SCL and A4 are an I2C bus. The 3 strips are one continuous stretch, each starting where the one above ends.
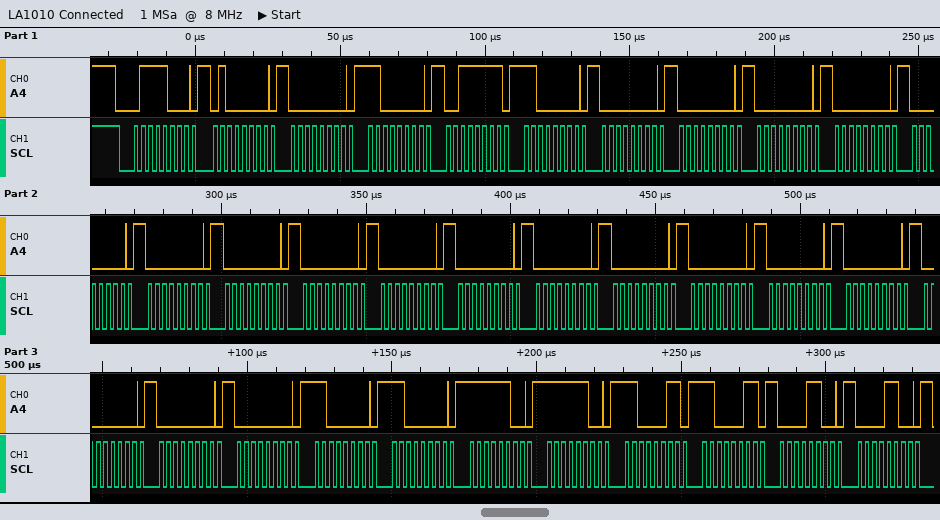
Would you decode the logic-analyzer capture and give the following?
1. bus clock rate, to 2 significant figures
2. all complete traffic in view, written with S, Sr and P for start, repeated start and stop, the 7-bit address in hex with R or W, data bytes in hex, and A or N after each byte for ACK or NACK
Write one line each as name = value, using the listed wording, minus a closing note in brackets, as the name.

bus clock rate, to 2 significant figures = 400 kHz
all complete traffic in view, written with S, Sr and P for start, repeated start and stop, the 7-bit address in hex with R or W, data bytes in hex, and A or N after each byte for ACK or NACK = S 3CW A 40 A 00 A C0 A 3F A C0 A 00 A 00 A 00 A 00 A 00 A 00 A 00 A 00 A 00 A 00 A 00 A 00 A 00 A 00 A 00 A 00 A 00 A 00 A C0 A C0 A FC A FC A C3 A C3 A 0C A 0C A
